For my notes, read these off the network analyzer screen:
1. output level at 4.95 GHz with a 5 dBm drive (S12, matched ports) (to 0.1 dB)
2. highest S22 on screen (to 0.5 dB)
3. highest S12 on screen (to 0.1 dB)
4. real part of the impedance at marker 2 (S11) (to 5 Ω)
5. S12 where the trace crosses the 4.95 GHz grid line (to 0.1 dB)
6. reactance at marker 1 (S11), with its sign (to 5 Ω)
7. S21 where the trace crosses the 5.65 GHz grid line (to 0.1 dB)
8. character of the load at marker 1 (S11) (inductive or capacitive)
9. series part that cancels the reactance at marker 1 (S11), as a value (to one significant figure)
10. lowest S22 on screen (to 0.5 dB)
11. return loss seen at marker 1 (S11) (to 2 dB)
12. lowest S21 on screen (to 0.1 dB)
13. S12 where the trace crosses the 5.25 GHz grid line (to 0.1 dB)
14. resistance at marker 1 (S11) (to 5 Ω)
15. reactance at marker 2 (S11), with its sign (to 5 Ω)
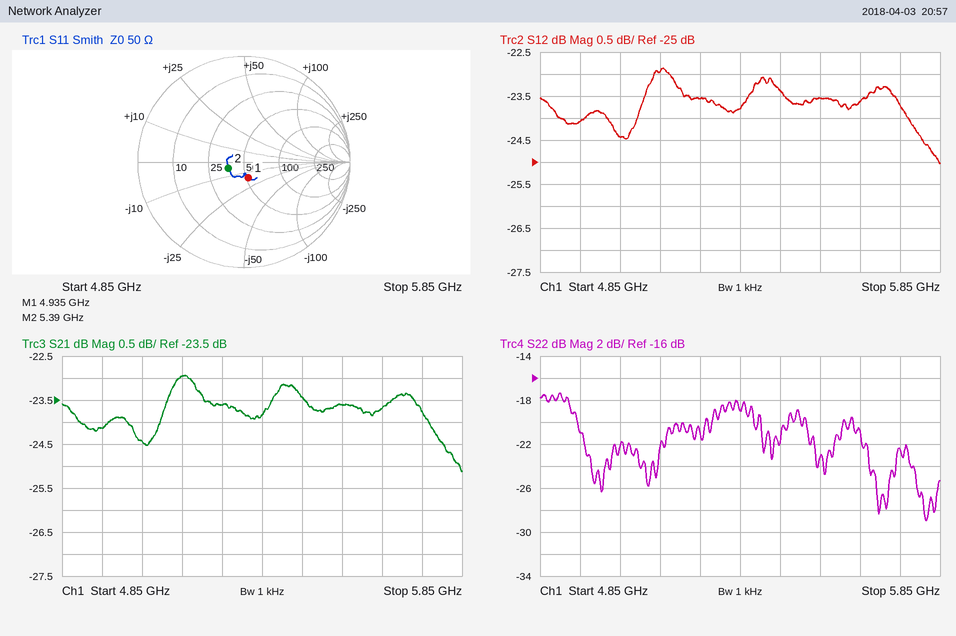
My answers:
-19.1 dBm
-17.5 dB
-22.9 dB
35 Ω
-24.1 dB
-15 Ω
-23.7 dB
capacitive
500 pH
-29.0 dB
16 dB
-25.1 dB
-23.6 dB
50 Ω
-5 Ω
